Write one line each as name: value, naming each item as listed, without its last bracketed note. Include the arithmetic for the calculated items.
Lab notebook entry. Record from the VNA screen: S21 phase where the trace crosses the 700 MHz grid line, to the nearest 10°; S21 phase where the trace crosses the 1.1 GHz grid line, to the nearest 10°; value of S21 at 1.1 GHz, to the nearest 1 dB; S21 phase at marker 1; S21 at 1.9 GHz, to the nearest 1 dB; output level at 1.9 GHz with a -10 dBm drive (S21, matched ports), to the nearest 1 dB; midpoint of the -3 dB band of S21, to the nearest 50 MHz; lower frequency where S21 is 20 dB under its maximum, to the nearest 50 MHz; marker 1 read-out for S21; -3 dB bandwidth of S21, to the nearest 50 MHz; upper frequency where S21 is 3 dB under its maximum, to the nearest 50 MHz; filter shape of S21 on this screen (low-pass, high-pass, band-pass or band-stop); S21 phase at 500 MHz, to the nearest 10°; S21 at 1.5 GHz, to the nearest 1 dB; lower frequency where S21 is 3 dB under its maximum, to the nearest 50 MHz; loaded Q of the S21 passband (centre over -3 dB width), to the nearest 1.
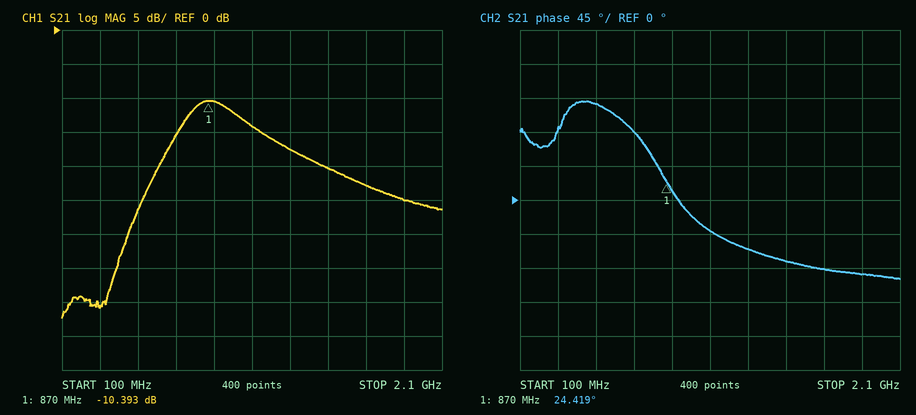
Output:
S21 phase where the trace crosses the 700 MHz grid line, to the nearest 10°: 90°
S21 phase where the trace crosses the 1.1 GHz grid line, to the nearest 10°: -40°
value of S21 at 1.1 GHz, to the nearest 1 dB: -14 dB
S21 phase at marker 1: 24.419°
S21 at 1.9 GHz, to the nearest 1 dB: -25 dB
output level at 1.9 GHz with a -10 dBm drive (S21, matched ports), to the nearest 1 dB: -10 dBm + (-25 dB) = -35 dBm
midpoint of the -3 dB band of S21, to the nearest 50 MHz: 900 MHz
lower frequency where S21 is 20 dB under its maximum, to the nearest 50 MHz: 450 MHz
marker 1 read-out for S21: -10.393 dB
-3 dB bandwidth of S21, to the nearest 50 MHz: 1.05 GHz − 750 MHz = 300 MHz
upper frequency where S21 is 3 dB under its maximum, to the nearest 50 MHz: 1.05 GHz
filter shape of S21 on this screen: band-pass
S21 phase at 500 MHz, to the nearest 10°: 130°
S21 at 1.5 GHz, to the nearest 1 dB: -20 dB
lower frequency where S21 is 3 dB under its maximum, to the nearest 50 MHz: 750 MHz
loaded Q of the S21 passband (centre over -3 dB width), to the nearest 1: 900 MHz / 300 MHz ≈ 3
